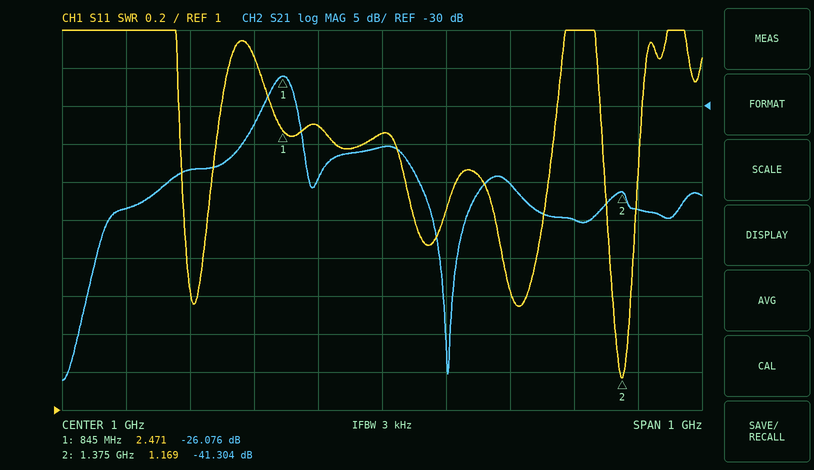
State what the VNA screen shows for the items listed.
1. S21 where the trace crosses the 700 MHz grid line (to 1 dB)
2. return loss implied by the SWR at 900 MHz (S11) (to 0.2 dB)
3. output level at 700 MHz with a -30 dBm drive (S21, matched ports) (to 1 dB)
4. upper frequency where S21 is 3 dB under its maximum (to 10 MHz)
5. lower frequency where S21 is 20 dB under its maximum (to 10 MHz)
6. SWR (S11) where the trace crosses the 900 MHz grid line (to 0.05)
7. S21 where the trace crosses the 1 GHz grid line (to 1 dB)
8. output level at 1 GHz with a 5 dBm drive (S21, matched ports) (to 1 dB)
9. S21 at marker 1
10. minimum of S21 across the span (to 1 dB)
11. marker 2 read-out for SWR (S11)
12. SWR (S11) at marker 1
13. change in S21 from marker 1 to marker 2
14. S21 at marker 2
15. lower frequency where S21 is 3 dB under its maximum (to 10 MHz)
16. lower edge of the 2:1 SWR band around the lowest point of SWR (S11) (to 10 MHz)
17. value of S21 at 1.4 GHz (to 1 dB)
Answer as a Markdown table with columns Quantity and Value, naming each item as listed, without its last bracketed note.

| Quantity | Value |
|---|---|
| S21 where the trace crosses the 700 MHz grid line | -38 dB |
| return loss implied by the SWR at 900 MHz (S11) | 7.4 dB |
| output level at 700 MHz with a -30 dBm drive (S21, matched ports) | -68 dBm |
| upper frequency where S21 is 3 dB under its maximum | 860 MHz |
| lower frequency where S21 is 20 dB under its maximum | 570 MHz |
| SWR (S11) where the trace crosses the 900 MHz grid line | 2.50 |
| S21 where the trace crosses the 1 GHz grid line | -35 dB |
| output level at 1 GHz with a 5 dBm drive (S21, matched ports) | -30 dBm |
| S21 at marker 1 | -26.076 dB |
| minimum of S21 across the span | -66 dB |
| marker 2 read-out for SWR | 1.169 |
| SWR (S11) at marker 1 | 2.471 |
| change in S21 from marker 1 to marker 2 | -15.228 dB |
| S21 at marker 2 | -41.304 dB |
| lower frequency where S21 is 3 dB under its maximum | 820 MHz |
| lower edge of the 2:1 SWR band around the lowest point of SWR (S11) | 1.35 GHz |
| value of S21 at 1.4 GHz | -44 dB |
